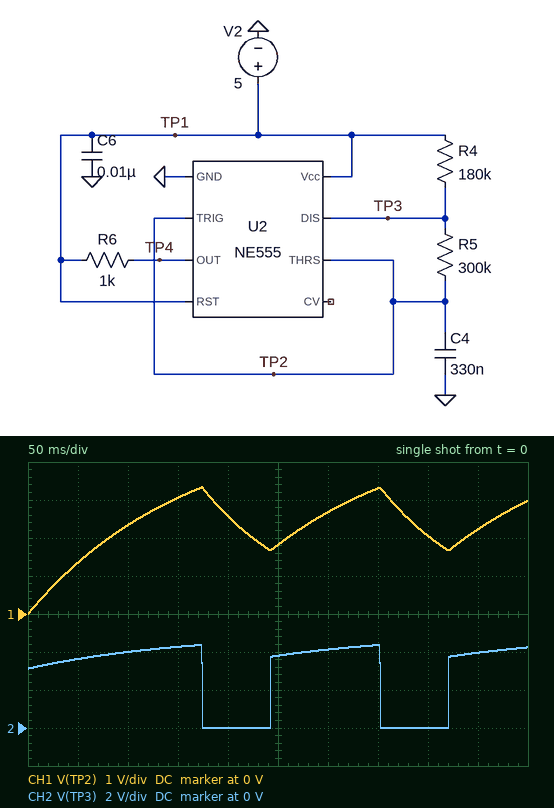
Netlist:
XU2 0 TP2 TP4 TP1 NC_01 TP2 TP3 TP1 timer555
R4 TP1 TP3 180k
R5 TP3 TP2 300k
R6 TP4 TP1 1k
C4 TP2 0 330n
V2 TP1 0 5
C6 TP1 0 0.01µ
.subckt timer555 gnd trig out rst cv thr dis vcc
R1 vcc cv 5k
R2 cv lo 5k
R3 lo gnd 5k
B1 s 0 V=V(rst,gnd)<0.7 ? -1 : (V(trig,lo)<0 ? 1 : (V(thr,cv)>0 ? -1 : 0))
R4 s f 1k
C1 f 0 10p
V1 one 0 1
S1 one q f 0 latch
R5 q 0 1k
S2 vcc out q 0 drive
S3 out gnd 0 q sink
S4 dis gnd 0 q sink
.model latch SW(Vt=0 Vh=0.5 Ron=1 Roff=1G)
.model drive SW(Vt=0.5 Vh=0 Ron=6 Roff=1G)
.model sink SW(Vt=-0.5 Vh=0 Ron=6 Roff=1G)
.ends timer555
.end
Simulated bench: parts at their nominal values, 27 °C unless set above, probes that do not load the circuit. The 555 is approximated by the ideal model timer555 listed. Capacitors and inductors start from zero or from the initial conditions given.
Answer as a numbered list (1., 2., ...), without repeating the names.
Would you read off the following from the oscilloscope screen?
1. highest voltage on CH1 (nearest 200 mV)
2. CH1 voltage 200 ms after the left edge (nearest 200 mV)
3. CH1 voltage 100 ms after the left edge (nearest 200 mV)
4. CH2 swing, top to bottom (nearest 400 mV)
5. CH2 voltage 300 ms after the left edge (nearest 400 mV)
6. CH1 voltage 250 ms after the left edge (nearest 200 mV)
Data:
1. 3.4 V
2. 2.6 V
3. 2.4 V
4. 4.4 V
5. 4.0 V
6. 1.8 V
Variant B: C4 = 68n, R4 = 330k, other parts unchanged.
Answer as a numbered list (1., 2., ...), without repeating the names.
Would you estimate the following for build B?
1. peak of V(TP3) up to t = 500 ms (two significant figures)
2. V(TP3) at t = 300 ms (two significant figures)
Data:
1. 4.1 V
2. 3.9 V
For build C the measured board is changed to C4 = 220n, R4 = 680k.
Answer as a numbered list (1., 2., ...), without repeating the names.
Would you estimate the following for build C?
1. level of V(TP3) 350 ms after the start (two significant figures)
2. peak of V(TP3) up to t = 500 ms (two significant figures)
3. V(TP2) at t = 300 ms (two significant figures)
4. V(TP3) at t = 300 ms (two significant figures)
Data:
1. 3.3 V
2. 3.8 V
3. 1.9 V
4. 2.9 V
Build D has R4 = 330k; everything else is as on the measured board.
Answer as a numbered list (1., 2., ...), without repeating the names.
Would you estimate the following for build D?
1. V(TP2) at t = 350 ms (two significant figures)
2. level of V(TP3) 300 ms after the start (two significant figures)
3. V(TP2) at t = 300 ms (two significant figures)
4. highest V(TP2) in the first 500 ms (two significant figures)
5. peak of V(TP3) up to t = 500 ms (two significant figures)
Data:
1. 2.4 V
2. 3.3 V
3. 1.7 V
4. 3.3 V
5. 4.1 V
